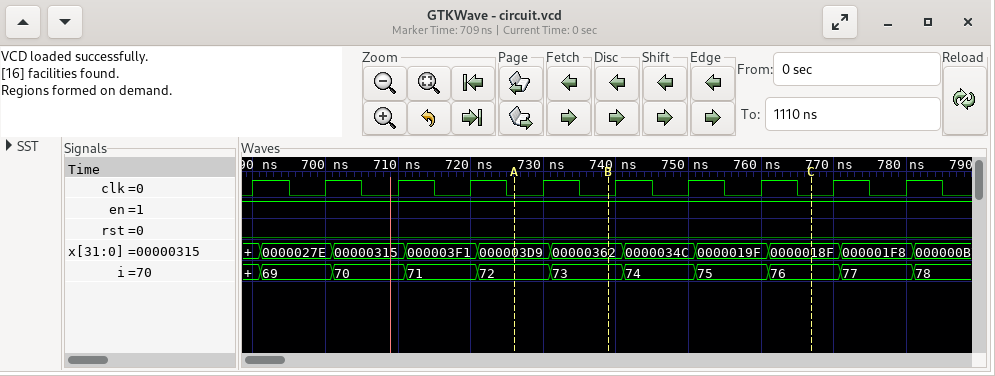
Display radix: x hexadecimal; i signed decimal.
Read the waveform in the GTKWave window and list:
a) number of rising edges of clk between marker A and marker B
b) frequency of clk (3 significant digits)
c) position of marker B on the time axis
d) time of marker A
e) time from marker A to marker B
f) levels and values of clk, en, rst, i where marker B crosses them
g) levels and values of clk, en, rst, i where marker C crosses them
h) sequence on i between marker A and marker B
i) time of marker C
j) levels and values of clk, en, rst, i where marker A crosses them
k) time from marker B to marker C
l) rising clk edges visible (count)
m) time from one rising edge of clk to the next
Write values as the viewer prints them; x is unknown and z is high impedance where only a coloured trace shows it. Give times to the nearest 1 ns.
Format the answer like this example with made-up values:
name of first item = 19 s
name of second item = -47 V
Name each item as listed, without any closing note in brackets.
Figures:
number of rising edges of clk between marker A and marker B = 1
frequency of clk = 100 MHz
position of marker B on the time axis = 739 ns
time of marker A = 726 ns
time from marker A to marker B = 13 ns
levels and values of clk, en, rst, i where marker B crosses them = clk=0, en=1, rst=0, i=73
levels and values of clk, en, rst, i where marker C crosses them = clk=0, en=1, rst=0, i=76
sequence on i between marker A and marker B = 72, 73
time of marker C = 767 ns
levels and values of clk, en, rst, i where marker A crosses them = clk=0, en=1, rst=0, i=72
time from marker B to marker C = 28 ns
rising clk edges visible = 10
time from one rising edge of clk to the next = 10 ns
